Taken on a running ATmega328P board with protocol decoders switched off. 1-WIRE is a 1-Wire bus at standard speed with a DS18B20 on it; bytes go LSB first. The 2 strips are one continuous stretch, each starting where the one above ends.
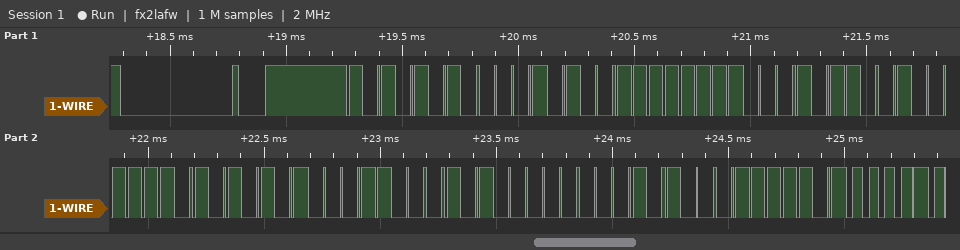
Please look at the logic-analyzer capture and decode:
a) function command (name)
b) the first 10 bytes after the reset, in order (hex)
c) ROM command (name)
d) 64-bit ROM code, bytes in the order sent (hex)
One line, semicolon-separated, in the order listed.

Read Scratchpad; 55 28 FF 68 F2 AA 18 05 28 BE; Match ROM; 28 FF 68 F2 AA 18 05 28
